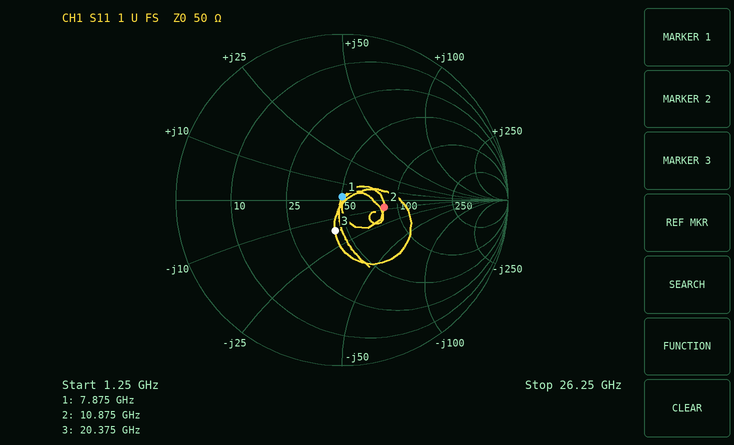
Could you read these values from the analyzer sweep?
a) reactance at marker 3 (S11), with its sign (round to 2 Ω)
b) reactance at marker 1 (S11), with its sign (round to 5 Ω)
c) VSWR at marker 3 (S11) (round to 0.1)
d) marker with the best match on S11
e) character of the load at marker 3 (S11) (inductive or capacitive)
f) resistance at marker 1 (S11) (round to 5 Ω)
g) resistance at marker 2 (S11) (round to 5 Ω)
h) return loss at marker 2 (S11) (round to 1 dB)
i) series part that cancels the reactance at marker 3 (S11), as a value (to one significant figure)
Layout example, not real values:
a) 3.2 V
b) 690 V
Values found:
a) -16 Ω
b) 0 Ω
c) 1.5
d) marker 1
e) capacitive
f) 50 Ω
g) 85 Ω
h) 12 dB
i) 100 pH
